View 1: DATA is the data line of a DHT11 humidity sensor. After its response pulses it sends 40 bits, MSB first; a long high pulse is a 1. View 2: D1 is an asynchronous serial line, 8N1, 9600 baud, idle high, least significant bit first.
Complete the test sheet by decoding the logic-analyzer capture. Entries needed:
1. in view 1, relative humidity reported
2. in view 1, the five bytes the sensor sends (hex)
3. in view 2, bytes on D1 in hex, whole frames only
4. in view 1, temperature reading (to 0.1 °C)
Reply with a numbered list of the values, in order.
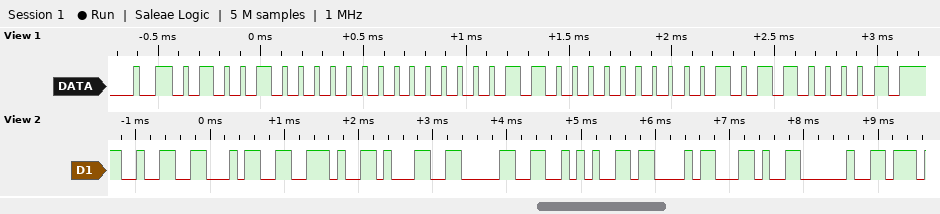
1. 72 %
2. 48 00 18 01 61
3. 32 34 2E 31 30 2A 43 2C 20
4. 24.1 °C
